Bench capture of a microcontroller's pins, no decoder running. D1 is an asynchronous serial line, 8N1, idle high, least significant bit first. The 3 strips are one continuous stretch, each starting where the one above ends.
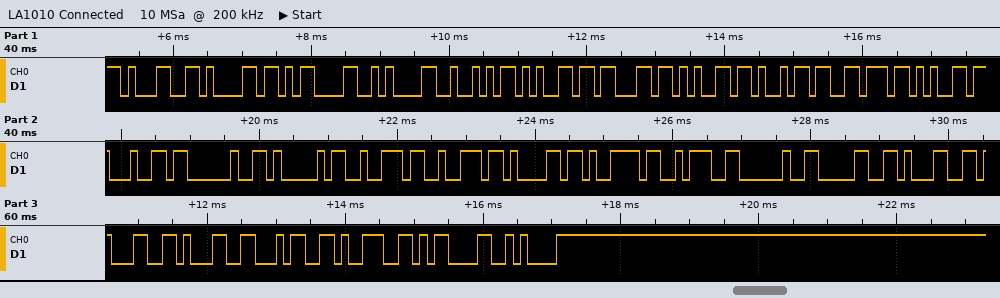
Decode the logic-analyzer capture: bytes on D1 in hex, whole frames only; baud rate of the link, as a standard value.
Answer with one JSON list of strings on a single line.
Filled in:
["31 61 0D 0A 52 65 63 65 69 76 65 64 20 41 72 72 61 79 3A 20 30 31 31 31 34 39 0D 0A", "9600 baud"]
